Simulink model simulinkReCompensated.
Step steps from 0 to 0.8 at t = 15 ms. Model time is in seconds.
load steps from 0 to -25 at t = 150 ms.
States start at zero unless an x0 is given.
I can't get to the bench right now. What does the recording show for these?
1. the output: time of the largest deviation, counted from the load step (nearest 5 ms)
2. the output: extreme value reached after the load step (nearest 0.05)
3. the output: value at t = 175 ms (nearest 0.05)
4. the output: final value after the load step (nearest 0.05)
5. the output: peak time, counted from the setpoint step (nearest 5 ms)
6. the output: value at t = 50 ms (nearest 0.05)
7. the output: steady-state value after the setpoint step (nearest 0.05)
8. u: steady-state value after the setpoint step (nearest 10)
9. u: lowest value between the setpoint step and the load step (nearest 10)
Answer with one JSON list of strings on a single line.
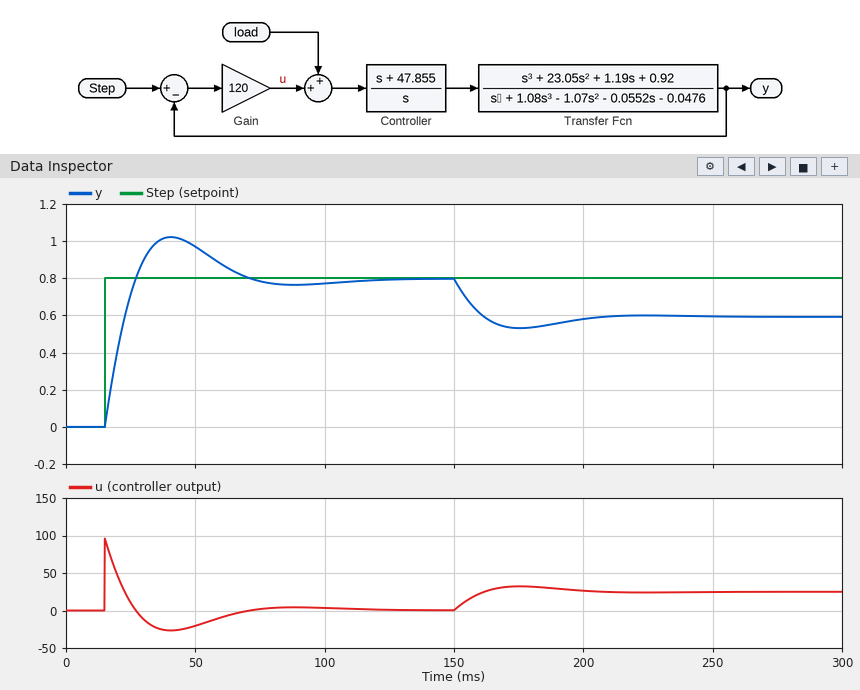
["25 ms", "0.55", "0.55", "0.60", "25 ms", "0.95", "0.80", "0", "-30"]
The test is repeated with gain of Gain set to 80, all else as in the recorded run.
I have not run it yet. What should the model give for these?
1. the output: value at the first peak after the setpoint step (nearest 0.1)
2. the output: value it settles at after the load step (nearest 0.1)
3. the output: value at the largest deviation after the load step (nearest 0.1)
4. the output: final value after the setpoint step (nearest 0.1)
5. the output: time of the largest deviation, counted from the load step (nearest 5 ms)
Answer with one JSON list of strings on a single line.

["1.1", "0.5", "0.4", "0.8", "35 ms"]
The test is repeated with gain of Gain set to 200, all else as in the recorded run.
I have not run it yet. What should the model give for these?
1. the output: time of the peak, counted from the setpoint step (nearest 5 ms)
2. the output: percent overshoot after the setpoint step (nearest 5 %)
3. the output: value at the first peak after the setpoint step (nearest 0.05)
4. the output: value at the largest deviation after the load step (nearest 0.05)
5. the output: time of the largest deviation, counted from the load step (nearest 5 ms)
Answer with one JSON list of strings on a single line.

["20 ms", "20 %", "0.95", "0.65", "20 ms"]
